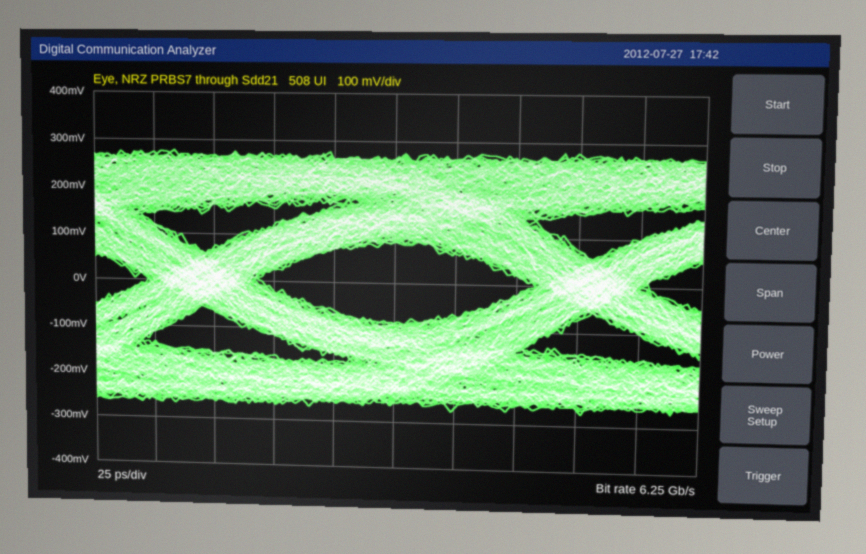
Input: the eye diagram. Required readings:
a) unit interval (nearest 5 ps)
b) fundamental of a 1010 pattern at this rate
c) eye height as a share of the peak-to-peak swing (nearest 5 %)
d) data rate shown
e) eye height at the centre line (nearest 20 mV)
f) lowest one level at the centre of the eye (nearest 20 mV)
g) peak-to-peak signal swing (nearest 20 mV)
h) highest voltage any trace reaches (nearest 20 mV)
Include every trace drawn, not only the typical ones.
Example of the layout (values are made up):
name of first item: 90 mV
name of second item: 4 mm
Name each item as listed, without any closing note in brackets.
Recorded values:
unit interval: 160 ps
fundamental of a 1010 pattern at this rate: 3.125 GHz
eye height as a share of the peak-to-peak swing: 30 %
data rate shown: 6.25 Gb/s
eye height at the centre line: 180 mV
lowest one level at the centre of the eye: 80 mV
peak-to-peak signal swing: 560 mV
highest voltage any trace reaches: 280 mV
